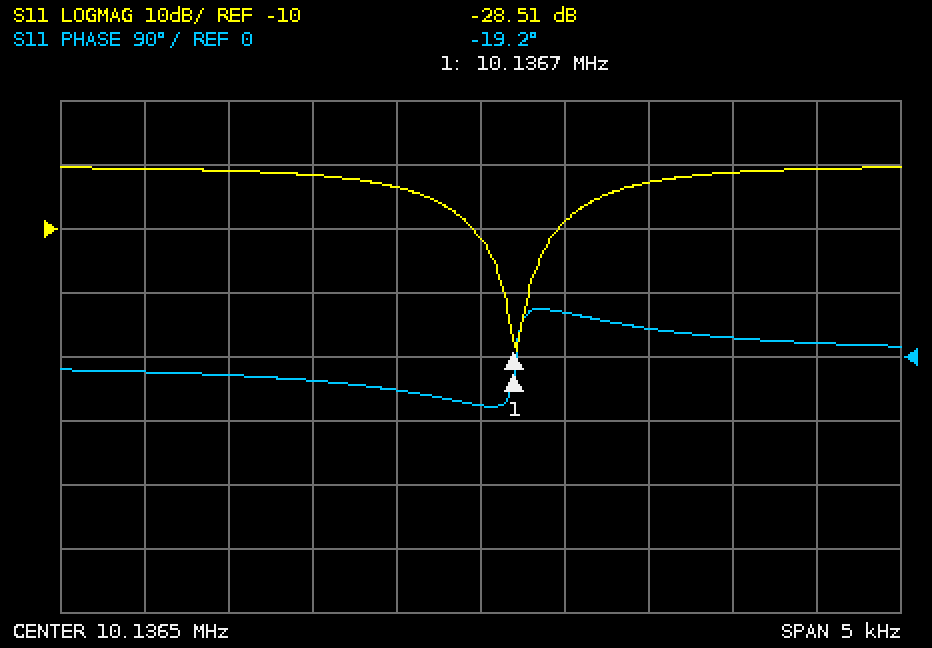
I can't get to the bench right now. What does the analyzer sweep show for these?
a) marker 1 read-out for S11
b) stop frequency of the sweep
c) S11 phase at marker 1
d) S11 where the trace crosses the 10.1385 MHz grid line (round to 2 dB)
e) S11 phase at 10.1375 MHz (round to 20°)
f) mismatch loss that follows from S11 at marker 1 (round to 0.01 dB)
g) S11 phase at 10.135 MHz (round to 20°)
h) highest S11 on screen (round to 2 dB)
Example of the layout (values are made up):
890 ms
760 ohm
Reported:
-28.51 dB
10.139 MHz
-19.2°
0 dB
40°
0.01 dB
-20°
0 dB
